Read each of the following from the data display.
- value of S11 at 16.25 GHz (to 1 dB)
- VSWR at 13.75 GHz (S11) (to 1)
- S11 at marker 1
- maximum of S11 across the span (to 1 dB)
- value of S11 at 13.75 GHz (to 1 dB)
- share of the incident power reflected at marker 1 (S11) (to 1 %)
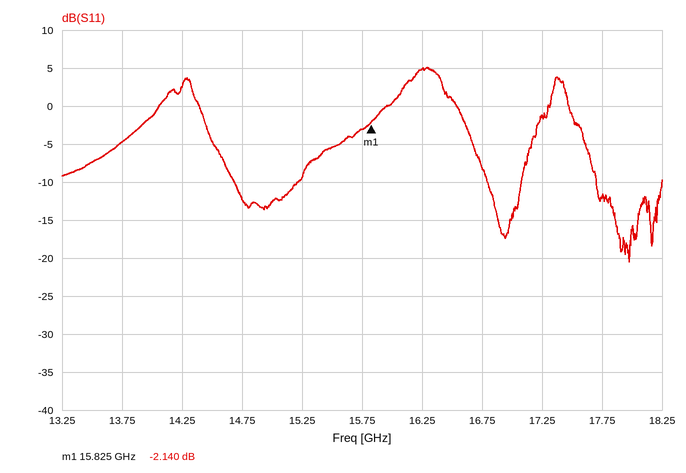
5 dB
4
-2.140 dB
5 dB
-5 dB
61 %
